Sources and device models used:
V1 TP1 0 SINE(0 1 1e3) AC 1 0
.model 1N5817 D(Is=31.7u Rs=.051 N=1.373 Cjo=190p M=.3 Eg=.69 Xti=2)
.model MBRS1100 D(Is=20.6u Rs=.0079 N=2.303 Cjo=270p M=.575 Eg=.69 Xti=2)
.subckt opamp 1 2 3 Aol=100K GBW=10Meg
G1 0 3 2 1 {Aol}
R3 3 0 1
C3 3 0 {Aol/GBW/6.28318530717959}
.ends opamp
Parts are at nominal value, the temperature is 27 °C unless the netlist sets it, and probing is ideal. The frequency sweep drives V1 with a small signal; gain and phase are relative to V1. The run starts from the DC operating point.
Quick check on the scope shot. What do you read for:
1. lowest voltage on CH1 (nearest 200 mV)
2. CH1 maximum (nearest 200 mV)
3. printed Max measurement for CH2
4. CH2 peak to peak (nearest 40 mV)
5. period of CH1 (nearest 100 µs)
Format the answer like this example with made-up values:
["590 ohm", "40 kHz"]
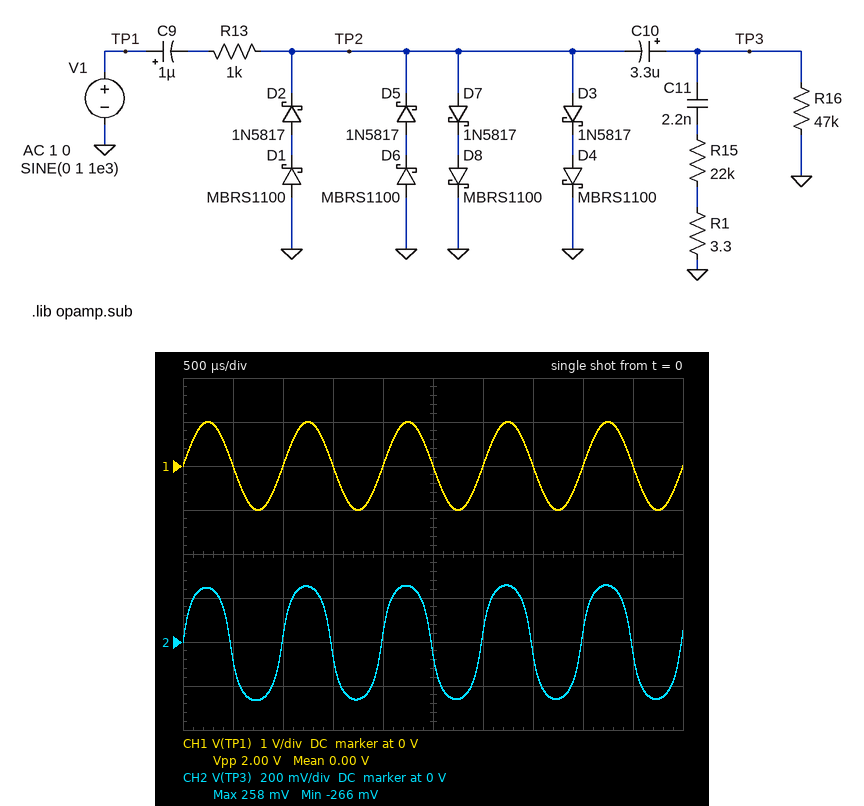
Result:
["-1.0 V", "1.0 V", "258 mV", "520 mV", "1.0 ms"]
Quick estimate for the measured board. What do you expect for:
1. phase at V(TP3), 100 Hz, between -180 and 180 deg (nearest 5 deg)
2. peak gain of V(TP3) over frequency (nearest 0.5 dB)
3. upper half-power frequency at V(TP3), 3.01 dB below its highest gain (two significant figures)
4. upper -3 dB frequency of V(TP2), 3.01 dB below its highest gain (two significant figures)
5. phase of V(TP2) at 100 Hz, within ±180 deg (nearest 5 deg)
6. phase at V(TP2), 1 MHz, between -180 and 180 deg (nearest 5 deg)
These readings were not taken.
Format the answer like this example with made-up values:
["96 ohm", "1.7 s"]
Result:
["40 deg", "-6.0 dB", "510 kHz", "510 kHz", "40 deg", "-50 deg"]
